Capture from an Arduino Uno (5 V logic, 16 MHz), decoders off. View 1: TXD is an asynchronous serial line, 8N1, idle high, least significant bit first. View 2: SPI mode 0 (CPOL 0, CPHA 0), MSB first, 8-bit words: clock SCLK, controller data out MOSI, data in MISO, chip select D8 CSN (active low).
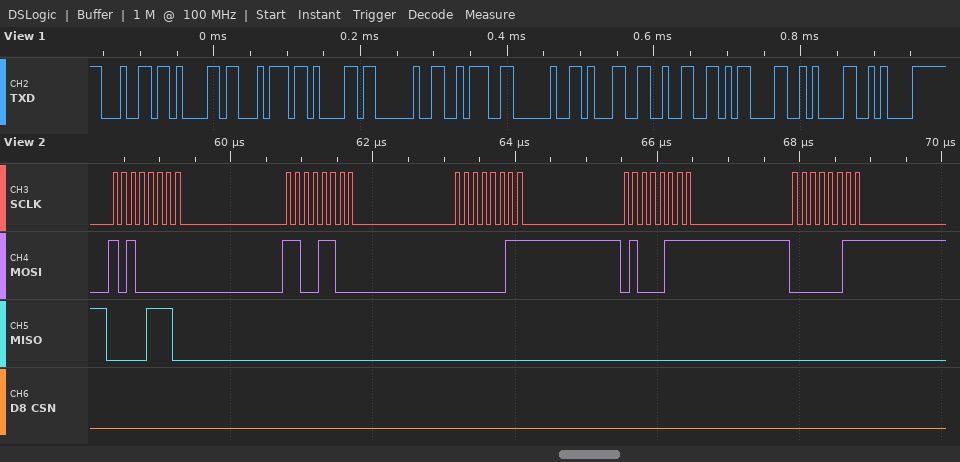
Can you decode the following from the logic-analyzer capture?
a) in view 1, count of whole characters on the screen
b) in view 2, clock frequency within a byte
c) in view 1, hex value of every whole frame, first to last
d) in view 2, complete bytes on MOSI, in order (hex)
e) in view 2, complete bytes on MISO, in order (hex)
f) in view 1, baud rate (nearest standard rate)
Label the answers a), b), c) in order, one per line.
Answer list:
a) 12
b) 8 MHz
c) 64 61 74 61 20 3A 20 31 32 0D 0A 0A
d) A0 CC 03 47 03
e) 0E 00 00 00 00
f) 115200 baud
